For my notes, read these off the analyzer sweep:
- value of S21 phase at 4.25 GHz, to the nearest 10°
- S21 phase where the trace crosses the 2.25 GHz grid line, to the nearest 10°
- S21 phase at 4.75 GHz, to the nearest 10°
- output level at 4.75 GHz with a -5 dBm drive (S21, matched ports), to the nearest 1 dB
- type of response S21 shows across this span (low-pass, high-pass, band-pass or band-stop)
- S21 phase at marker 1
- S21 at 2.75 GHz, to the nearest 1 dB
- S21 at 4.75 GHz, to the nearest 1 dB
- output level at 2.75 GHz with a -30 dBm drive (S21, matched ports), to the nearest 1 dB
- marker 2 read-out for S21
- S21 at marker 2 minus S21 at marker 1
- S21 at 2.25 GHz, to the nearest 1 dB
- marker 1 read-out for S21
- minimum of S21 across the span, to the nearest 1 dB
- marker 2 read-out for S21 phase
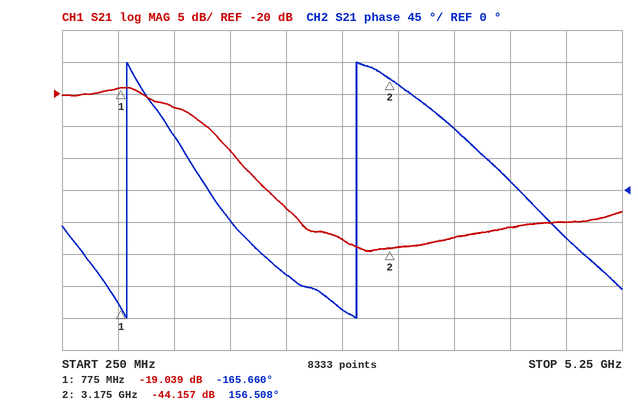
10°
-120°
-70°
-45 dBm
low-pass
-165.660°
-43 dB
-40 dB
-73 dBm
-44.157 dB
-25.118 dB
-38 dB
-19.039 dB
-45 dB
156.508°
